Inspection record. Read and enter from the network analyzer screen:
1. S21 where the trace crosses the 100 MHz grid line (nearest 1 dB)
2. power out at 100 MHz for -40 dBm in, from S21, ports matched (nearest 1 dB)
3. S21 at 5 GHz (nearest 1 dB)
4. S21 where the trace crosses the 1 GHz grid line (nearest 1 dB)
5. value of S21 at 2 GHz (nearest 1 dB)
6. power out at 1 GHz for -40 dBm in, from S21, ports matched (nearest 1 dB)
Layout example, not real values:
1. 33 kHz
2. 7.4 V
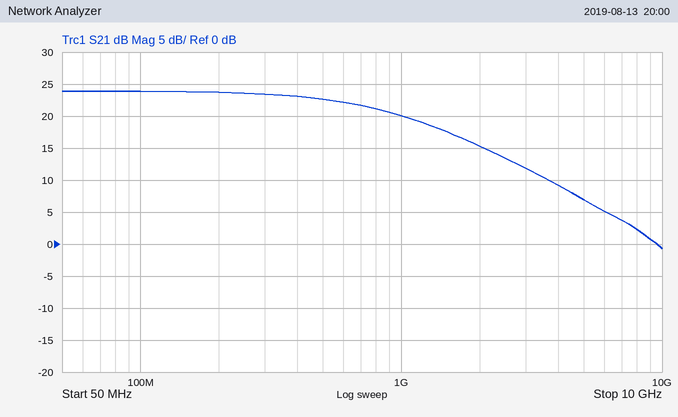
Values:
1. 24 dB
2. -16 dBm
3. 7 dB
4. 20 dB
5. 15 dB
6. -20 dBm
